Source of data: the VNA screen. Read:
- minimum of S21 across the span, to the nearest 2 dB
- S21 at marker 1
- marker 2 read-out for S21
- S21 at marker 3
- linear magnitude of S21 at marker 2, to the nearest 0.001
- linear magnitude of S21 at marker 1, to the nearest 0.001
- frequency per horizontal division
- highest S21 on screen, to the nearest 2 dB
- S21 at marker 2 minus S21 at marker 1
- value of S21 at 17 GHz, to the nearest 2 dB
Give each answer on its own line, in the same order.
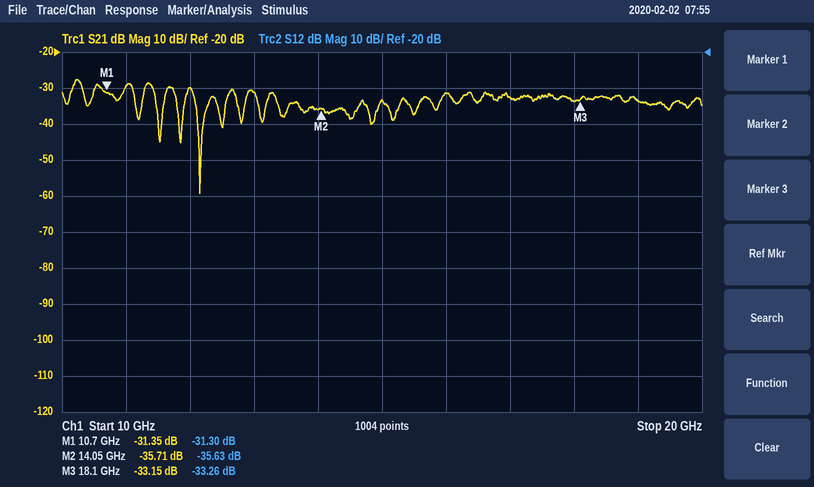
-60 dB
-31.35 dB
-35.71 dB
-33.15 dB
0.016
0.027
1 GHz
-28 dB
-4.36 dB
-32 dB
